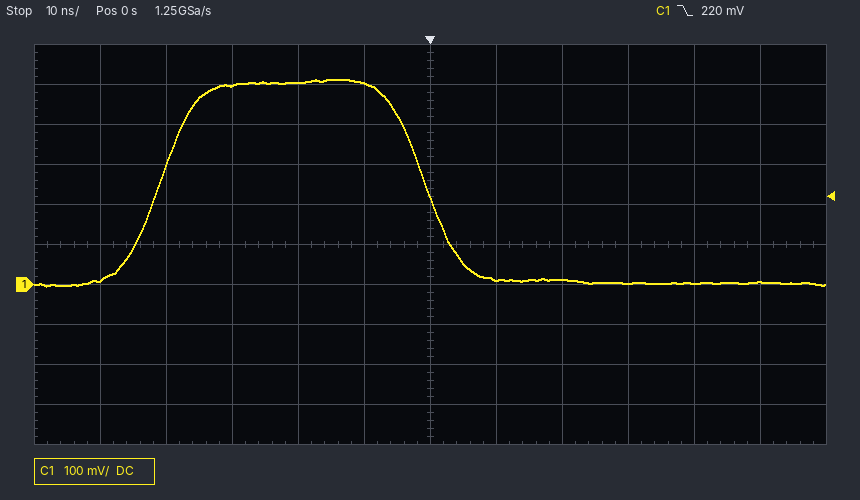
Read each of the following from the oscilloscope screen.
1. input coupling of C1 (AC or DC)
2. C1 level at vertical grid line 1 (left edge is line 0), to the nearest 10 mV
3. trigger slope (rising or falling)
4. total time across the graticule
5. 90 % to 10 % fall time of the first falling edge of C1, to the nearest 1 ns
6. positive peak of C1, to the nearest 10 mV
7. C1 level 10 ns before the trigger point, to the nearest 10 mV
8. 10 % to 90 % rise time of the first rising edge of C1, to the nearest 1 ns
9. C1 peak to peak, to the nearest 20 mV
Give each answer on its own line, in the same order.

DC
10 mV
falling
120 ns
11 ns
510 mV
500 mV
11 ns
520 mV
